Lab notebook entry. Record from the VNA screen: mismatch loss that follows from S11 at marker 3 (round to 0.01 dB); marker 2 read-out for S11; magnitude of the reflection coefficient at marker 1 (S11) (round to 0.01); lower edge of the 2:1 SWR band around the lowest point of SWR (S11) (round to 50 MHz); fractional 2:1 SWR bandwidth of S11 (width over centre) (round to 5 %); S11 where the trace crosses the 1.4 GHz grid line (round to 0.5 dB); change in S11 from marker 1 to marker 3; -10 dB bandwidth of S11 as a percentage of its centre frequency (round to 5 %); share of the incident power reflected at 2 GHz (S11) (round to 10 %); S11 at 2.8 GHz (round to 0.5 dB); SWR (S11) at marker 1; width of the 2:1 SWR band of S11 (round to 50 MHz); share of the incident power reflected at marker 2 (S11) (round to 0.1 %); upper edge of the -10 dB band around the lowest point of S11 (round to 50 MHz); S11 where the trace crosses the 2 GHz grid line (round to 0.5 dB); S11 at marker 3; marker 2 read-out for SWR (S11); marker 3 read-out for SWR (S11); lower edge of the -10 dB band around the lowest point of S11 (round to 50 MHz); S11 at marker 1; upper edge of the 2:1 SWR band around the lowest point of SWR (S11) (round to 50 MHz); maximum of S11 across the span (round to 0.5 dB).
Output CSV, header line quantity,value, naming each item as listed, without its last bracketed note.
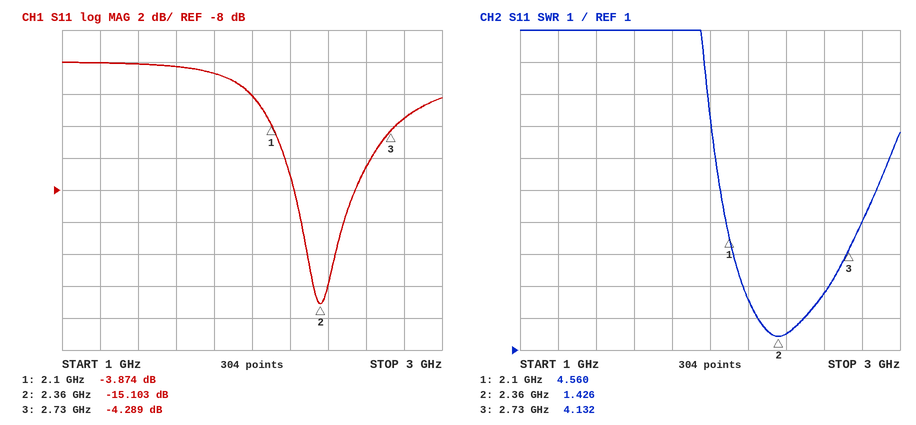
quantity,value
mismatch loss that follows from S11 at marker 3,2.02 dB
marker 2 read-out for S11,-15.103 dB
magnitude of the reflection coefficient at marker 1 (S11),0.64
lower edge of the 2:1 SWR band around the lowest point of SWR (S11),2.25 GHz
fractional 2:1 SWR bandwidth of S11 (width over centre),10 %
S11 where the trace crosses the 1.4 GHz grid line,0.0 dB
change in S11 from marker 1 to marker 3,-0.415 dB
-10 dB bandwidth of S11 as a percentage of its centre frequency,10 %
share of the incident power reflected at 2 GHz (S11),60 %
S11 at 2.8 GHz,-3.5 dB
SWR (S11) at marker 1,4.560
width of the 2:1 SWR band of S11,250 MHz
share of the incident power reflected at marker 2 (S11),3.1 %
upper edge of the -10 dB band around the lowest point of S11,2.50 GHz
S11 where the trace crosses the 2 GHz grid line,-2.0 dB
S11 at marker 3,-4.289 dB
marker 2 read-out for SWR,1.426
marker 3 read-out for SWR,4.132
lower edge of the -10 dB band around the lowest point of S11,2.25 GHz
S11 at marker 1,-3.874 dB
upper edge of the 2:1 SWR band around the lowest point of SWR (S11),2.50 GHz
maximum of S11 across the span,0.0 dB
